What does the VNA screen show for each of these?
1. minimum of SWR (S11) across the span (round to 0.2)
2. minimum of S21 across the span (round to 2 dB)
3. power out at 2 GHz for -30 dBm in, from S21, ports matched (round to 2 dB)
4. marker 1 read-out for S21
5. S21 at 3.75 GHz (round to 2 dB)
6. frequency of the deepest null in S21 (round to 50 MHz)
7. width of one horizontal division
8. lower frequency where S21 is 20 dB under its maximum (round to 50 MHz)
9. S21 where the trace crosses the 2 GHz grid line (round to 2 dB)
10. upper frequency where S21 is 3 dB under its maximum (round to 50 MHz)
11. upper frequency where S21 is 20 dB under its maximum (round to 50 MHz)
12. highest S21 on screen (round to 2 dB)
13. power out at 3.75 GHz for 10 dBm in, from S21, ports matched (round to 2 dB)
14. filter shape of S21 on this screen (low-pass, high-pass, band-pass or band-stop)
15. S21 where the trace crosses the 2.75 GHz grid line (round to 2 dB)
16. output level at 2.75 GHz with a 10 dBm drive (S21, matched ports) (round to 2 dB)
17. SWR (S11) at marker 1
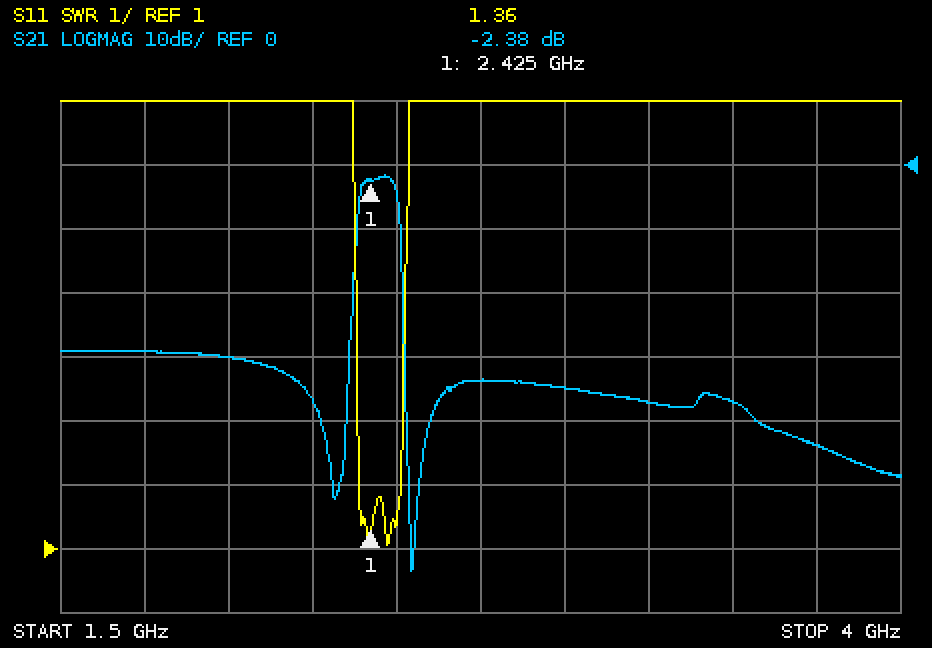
1.0
-64 dB
-60 dBm
-2.38 dB
-44 dB
2.55 GHz
250 MHz
2.35 GHz
-30 dB
2.50 GHz
2.50 GHz
-2 dB
-34 dBm
band-pass
-34 dB
-24 dBm
1.36
